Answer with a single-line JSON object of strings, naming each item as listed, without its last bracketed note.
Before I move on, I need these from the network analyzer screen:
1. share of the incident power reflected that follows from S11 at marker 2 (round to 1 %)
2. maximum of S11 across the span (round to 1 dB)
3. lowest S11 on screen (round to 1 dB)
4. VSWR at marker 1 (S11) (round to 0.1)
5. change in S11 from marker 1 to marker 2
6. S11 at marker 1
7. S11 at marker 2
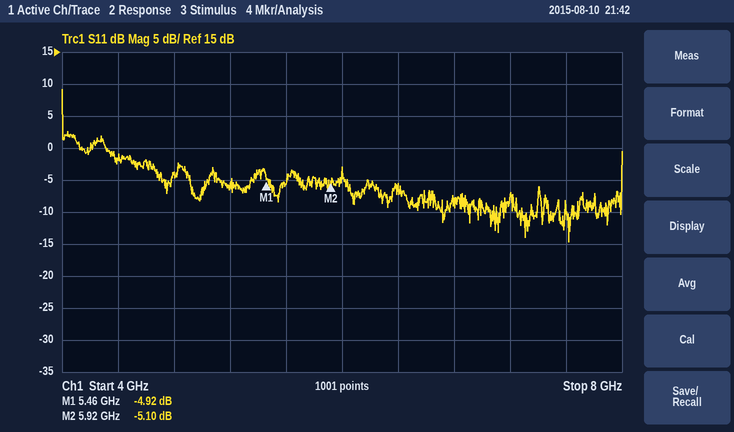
{"share of the incident power reflected that follows from S11 at marker 2": "31 %", "maximum of S11 across the span": "9 dB", "lowest S11 on screen": "-15 dB", "VSWR at marker 1 (S11)": "3.6", "change in S11 from marker 1 to marker 2": "-0.18 dB", "S11 at marker 1": "-4.92 dB", "S11 at marker 2": "-5.10 dB"}
